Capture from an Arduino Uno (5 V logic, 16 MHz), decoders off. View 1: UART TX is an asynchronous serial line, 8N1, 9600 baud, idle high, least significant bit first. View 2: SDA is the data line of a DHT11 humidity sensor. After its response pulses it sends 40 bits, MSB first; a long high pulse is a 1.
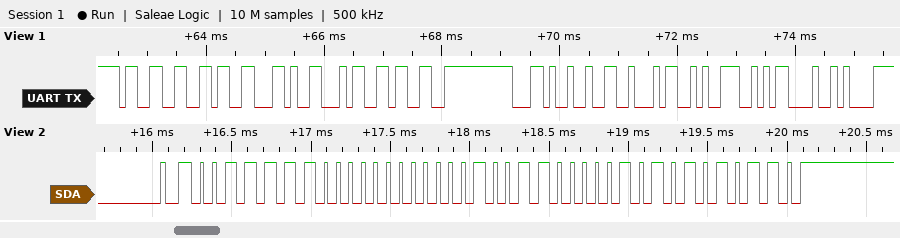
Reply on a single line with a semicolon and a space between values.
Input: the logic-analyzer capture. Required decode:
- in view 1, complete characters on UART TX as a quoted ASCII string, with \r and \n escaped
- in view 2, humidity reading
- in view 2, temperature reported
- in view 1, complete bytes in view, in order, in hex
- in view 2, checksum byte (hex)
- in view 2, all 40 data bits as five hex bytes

"36,43,249\r\n"; 62 %; 19.5 °C; 33 36 2C 34 33 2C 32 34 39 0D 0A; 0x56; 3E 00 13 05 56
